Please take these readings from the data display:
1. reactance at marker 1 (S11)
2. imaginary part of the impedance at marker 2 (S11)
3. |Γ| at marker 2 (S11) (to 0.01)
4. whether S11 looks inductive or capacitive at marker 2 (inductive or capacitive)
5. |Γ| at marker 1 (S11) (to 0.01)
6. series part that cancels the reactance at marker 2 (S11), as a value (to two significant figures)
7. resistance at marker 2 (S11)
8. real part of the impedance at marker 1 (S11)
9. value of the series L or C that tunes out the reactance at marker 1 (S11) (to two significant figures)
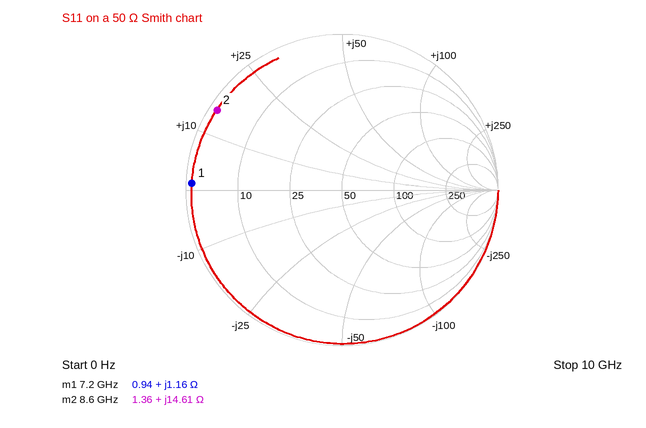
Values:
+1.16 Ω
+14.61 Ω
0.95
inductive
0.96
1.3 pF
1.36 Ω
0.94 Ω
19 pF
